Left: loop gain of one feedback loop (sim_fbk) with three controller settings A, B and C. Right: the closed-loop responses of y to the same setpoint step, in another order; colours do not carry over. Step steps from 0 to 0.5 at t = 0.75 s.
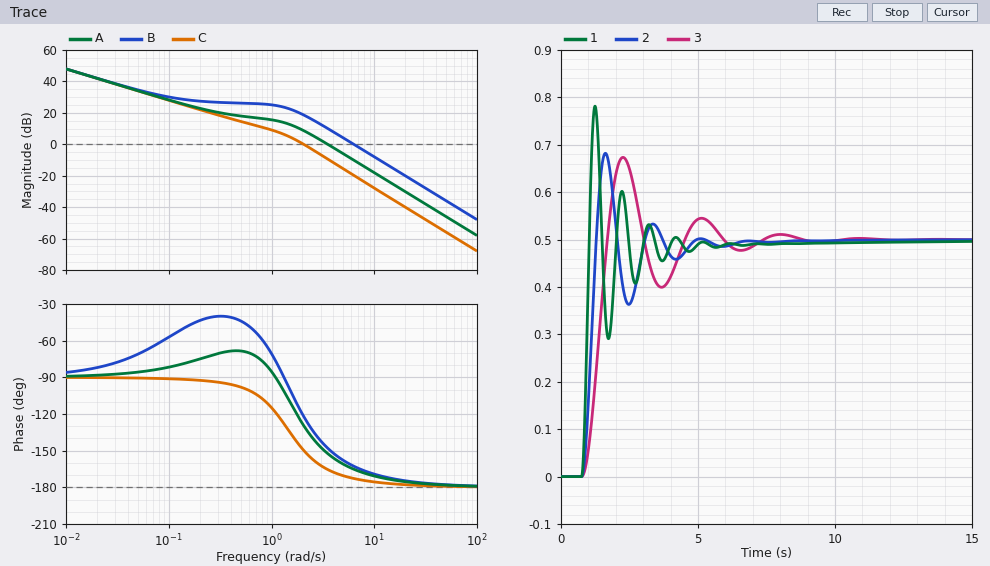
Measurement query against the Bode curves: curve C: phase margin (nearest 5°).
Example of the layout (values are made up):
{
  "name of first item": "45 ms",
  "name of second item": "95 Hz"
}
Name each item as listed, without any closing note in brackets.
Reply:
{
  "curve C: phase margin": "30°"
}
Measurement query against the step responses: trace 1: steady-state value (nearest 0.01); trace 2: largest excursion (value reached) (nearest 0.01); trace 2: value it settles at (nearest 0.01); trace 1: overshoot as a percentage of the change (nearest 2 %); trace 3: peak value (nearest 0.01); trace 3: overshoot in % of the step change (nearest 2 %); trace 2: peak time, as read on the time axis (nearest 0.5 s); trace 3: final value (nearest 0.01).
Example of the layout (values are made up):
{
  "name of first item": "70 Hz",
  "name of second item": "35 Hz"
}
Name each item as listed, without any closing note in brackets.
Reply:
{
  "trace 1: steady-state value": "0.50",
  "trace 2: largest excursion (value reached)": "0.68",
  "trace 2: value it settles at": "0.50",
  "trace 1: overshoot as a percentage of the change": "56 %",
  "trace 3: peak value": "0.67",
  "trace 3: overshoot in % of the step change": "34 %",
  "trace 2: peak time, as read on the time axis": "1.5 s",
  "trace 3: final value": "0.50"
}
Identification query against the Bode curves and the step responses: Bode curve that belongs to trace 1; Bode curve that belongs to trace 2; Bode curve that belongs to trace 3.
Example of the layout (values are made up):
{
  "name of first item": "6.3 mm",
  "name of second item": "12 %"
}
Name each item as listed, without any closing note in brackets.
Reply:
{
  "Bode curve that belongs to trace 1": "B",
  "Bode curve that belongs to trace 2": "A",
  "Bode curve that belongs to trace 3": "C"
}
